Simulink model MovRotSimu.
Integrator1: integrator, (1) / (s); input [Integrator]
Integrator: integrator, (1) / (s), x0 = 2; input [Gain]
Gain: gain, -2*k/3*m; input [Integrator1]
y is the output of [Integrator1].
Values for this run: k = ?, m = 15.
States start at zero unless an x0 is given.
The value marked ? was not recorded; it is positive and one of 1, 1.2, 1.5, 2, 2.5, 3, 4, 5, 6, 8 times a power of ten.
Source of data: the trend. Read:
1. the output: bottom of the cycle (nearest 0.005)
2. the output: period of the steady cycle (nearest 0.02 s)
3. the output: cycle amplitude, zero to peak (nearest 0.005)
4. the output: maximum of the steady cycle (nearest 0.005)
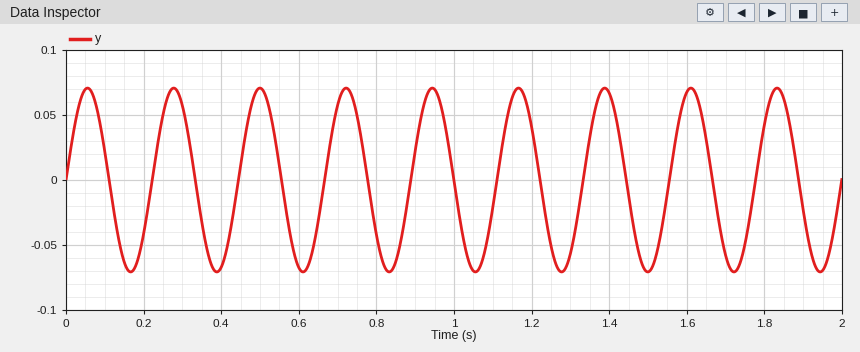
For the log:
-0.070
0.22 s
0.070
0.070
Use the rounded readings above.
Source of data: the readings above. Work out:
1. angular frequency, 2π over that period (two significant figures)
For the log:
29 rad/s
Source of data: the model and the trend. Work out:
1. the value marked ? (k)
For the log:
80
